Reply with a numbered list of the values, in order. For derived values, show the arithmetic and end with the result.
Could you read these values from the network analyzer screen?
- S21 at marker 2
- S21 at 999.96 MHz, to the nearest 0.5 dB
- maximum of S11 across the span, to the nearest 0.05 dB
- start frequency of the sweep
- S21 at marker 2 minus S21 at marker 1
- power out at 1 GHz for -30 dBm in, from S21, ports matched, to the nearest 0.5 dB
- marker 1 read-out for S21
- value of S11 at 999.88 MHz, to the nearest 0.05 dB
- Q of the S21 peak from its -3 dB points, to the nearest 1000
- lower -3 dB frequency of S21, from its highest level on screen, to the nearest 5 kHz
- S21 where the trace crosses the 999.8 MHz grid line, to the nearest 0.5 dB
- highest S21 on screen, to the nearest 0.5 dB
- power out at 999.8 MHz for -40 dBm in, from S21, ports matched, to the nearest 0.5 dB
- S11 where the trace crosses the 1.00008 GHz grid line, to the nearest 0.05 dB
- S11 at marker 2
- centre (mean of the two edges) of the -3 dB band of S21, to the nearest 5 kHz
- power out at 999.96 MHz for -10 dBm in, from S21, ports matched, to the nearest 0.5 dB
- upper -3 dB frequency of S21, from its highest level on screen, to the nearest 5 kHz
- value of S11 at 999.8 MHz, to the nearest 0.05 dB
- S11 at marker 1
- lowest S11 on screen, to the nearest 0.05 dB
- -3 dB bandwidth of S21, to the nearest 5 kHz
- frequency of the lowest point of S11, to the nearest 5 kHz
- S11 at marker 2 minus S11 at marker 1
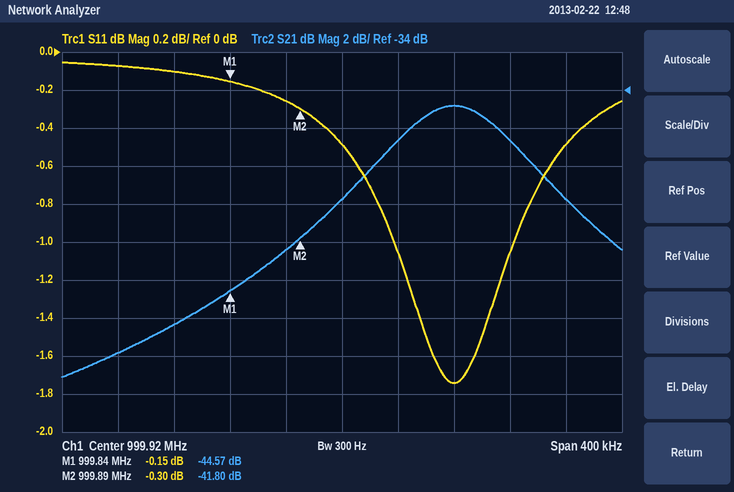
1. -41.80 dB
2. -36.5 dB
3. -0.05 dB
4. 999.72 MHz
5. -41.8 − (-44.57) = 2.77 dB
6. -30 dBm + (-35.0 dB) = -65.0 dBm
7. -44.57 dB
8. -0.25 dB
9. 1 GHz / 110 kHz ≈ 9091, so 9000 to the nearest 1000
10. 999.945 MHz
11. -46.5 dB
12. -35.0 dB
13. -40 dBm + (-46.5 dB) = -86.5 dBm
14. -0.50 dB
15. -0.30 dB
16. 1.000000 GHz
17. -10 dBm + (-36.5 dB) = -46.5 dBm
18. 1.000055 GHz
19. -0.10 dB
20. -0.15 dB
21. -1.75 dB
22. 1.000055 GHz − 999.945 MHz = 110 kHz
23. 1.000000 GHz
24. -0.3 − (-0.15) = -0.15 dB
